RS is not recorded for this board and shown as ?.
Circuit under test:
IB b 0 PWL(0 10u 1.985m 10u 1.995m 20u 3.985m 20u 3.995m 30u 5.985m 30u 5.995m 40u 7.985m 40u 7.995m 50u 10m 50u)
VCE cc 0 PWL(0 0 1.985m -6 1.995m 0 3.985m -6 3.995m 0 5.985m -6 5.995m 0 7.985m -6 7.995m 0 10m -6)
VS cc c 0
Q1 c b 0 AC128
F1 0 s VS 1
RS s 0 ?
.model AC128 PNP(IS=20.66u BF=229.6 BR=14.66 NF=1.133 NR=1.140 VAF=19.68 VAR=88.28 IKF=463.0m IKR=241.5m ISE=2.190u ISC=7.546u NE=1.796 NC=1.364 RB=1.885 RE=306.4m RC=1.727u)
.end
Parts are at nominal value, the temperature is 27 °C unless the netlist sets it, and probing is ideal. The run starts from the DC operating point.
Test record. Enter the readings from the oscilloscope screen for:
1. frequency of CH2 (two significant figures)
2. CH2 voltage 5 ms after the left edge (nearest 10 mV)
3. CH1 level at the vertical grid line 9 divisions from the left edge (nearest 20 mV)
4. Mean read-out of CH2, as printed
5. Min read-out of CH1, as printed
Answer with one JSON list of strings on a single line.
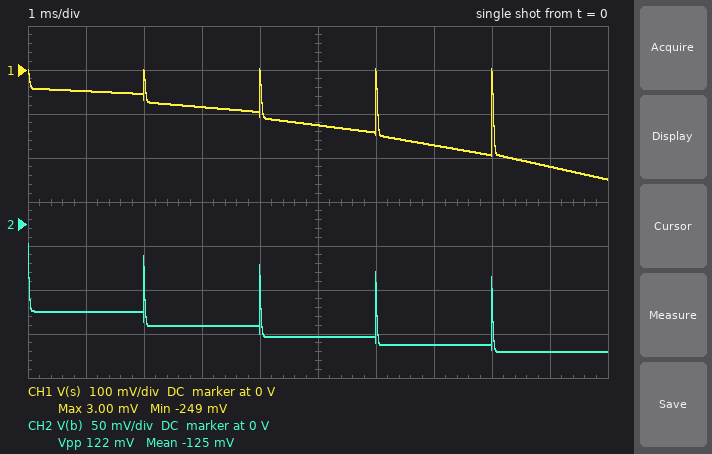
["500 Hz", "-130 mV", "-220 mV", "-125 mV", "-249 mV"]
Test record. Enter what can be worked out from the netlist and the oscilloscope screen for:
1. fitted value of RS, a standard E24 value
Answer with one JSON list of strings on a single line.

["68 Ω"]
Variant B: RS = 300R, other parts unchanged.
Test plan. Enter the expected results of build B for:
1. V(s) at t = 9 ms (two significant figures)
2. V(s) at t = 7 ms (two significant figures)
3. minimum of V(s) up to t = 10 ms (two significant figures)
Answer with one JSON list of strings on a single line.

["-970 mV", "-760 mV", "-1.1 V"]
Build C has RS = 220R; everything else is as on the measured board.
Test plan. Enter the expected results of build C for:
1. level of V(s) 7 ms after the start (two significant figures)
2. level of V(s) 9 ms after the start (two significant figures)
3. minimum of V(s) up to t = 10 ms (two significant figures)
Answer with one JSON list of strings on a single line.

["-550 mV", "-710 mV", "-810 mV"]
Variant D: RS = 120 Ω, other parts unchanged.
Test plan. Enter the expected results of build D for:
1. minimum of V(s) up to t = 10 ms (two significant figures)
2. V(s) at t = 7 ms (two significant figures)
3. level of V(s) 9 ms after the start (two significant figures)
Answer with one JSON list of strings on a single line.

["-440 mV", "-300 mV", "-390 mV"]
